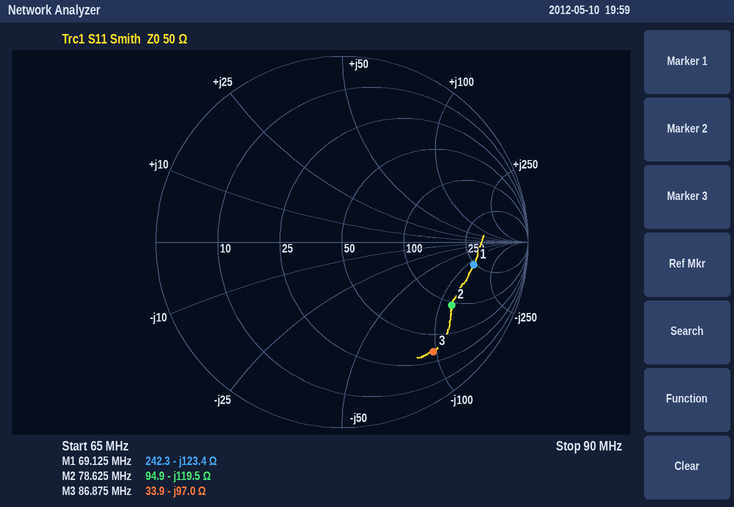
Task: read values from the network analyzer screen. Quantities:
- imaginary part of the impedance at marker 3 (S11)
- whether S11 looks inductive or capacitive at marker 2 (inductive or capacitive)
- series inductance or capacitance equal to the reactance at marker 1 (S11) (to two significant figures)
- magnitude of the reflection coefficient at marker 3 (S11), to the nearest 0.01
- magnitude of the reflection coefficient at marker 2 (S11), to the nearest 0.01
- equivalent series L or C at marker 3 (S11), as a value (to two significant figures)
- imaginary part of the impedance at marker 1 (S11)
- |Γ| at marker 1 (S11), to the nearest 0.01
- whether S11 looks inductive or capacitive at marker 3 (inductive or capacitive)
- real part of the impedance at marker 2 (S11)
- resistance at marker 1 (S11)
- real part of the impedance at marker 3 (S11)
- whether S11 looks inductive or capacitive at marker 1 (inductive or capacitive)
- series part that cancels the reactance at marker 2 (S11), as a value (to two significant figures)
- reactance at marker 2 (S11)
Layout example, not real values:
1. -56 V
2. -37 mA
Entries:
1. -97.0 Ω
2. capacitive
3. 19 pF
4. 0.77
5. 0.68
6. 19 pF
7. -123.4 Ω
8. 0.72
9. capacitive
10. 94.9 Ω
11. 242.3 Ω
12. 33.9 Ω
13. capacitive
14. 240 nH
15. -119.5 Ω
